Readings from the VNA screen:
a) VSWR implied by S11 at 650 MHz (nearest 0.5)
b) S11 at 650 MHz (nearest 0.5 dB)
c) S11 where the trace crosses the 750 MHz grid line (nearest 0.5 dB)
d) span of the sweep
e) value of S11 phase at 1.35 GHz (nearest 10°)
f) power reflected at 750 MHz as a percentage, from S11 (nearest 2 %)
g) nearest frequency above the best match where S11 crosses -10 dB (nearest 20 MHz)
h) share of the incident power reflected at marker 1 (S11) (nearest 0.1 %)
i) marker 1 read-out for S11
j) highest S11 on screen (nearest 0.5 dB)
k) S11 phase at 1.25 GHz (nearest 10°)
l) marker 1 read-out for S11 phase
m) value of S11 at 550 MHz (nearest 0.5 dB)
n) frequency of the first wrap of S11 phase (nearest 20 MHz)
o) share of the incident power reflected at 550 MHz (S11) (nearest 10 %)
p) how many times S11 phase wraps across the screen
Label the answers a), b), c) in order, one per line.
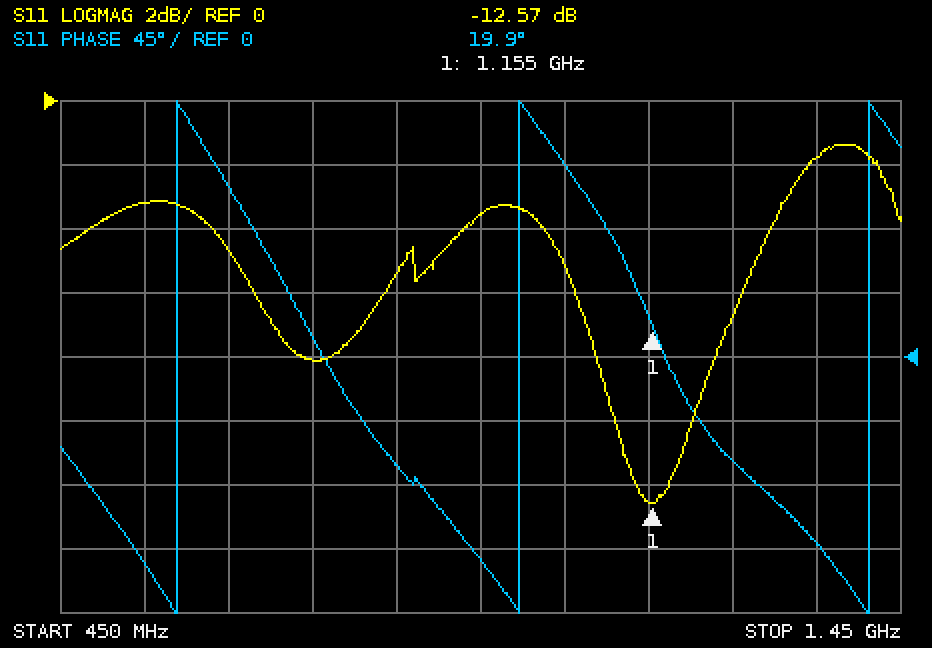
a) 4.0
b) -4.5 dB
c) -8.0 dB
d) 1 GHz
e) -130°
f) 16 %
g) 1.20 GHz
h) 5.5 %
i) -12.57 dB
j) -1.5 dB
k) -70°
l) 19.9°
m) -3.0 dB
n) 580 MHz
o) 50 %
p) 3
